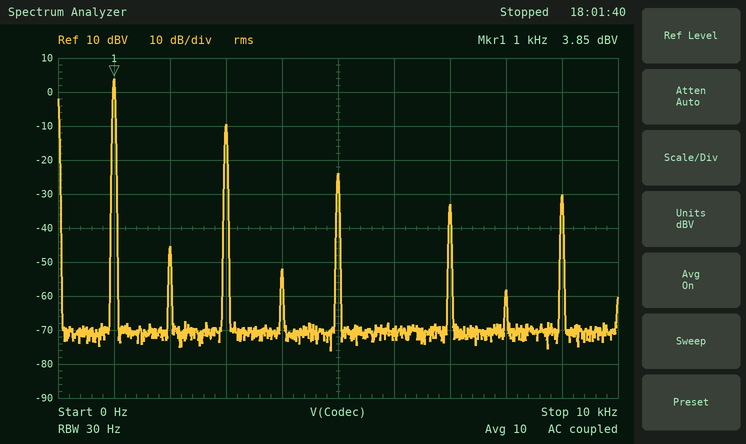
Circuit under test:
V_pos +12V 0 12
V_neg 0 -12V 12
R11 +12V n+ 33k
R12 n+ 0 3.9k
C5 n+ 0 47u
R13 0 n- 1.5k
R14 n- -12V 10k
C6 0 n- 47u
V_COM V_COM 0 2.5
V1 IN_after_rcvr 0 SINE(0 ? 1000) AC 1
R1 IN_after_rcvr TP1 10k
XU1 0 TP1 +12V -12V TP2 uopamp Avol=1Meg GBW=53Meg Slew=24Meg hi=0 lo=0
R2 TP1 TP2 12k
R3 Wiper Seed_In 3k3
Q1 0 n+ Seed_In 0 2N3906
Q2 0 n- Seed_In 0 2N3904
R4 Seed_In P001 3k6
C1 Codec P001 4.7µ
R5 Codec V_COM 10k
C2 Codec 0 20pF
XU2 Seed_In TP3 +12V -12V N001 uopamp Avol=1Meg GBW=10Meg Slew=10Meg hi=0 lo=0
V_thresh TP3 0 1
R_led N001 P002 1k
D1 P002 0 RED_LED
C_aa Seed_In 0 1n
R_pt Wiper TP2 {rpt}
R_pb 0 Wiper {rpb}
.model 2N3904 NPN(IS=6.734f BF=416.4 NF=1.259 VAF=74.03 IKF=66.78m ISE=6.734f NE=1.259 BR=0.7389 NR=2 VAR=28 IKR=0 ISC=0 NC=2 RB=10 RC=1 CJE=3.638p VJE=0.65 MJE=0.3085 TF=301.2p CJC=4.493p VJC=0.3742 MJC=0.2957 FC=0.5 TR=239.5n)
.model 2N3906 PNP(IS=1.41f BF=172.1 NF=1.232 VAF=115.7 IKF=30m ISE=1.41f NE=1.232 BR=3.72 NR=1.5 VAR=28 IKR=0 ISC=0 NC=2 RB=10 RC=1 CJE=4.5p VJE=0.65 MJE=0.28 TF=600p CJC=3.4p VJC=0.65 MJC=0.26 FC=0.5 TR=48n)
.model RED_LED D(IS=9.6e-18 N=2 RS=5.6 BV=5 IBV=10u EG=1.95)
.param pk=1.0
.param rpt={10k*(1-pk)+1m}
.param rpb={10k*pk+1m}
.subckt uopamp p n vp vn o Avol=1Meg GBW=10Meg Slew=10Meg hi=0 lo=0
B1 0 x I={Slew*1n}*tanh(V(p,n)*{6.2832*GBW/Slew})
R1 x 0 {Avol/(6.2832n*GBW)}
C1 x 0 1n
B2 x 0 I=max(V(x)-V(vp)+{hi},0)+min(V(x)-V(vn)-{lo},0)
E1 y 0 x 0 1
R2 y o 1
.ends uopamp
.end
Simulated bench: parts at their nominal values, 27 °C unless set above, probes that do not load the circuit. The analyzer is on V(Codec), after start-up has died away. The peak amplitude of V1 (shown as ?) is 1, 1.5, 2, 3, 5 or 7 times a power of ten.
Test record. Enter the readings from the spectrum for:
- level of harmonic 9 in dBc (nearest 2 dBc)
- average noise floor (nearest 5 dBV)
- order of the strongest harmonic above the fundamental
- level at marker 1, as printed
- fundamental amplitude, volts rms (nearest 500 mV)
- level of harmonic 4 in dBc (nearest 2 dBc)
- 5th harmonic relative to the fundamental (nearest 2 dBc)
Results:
-34 dBc
-70 dBV
3
3.85 dBV
1.5 V
-56 dBc
-28 dBc
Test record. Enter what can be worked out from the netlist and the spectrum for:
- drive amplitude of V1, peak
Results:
5 V
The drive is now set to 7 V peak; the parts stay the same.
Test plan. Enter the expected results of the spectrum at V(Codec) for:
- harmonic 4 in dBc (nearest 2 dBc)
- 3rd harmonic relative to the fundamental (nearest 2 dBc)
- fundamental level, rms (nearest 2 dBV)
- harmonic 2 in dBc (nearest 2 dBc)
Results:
-46 dBc
-12 dBc
4 dBV
-42 dBc
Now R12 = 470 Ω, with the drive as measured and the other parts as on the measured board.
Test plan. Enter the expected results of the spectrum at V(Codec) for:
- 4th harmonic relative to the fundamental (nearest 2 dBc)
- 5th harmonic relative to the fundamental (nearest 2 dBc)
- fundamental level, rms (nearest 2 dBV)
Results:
-22 dBc
-22 dBc
2 dBV
